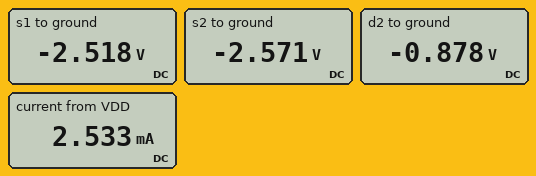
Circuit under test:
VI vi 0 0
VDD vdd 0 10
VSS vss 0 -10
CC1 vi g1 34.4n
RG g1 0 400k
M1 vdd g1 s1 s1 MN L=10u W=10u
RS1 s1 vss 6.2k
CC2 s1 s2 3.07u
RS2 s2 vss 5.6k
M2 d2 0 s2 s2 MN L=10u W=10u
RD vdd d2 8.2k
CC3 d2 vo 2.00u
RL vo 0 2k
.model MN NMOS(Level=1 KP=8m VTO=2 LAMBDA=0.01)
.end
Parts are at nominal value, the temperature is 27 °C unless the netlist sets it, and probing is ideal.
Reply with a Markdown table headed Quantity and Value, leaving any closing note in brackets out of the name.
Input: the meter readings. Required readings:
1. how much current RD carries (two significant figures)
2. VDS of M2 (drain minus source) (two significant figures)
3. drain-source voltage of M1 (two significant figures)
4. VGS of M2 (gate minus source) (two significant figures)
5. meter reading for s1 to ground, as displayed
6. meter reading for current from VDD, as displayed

| Quantity | Value |
|---|---|
| how much current RD carries | 1.3 mA |
| VDS of M2 (drain minus source) | 1.7 V |
| drain-source voltage of M1 | 13 V |
| VGS of M2 (gate minus source) | 2.6 V |
| meter reading for s1 to ground, as displayed | -2.518 V |
| meter reading for current from VDD, as displayed | 2.533 mA |
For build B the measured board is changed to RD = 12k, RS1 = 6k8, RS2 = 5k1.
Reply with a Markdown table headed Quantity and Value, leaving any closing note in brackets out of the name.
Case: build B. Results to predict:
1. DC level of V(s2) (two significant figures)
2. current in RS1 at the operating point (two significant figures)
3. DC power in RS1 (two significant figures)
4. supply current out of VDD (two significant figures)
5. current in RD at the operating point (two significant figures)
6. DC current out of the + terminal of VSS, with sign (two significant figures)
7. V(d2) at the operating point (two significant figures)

| Quantity | Value |
|---|---|
| DC level of V(s2) | -4.1 V |
| current in RS1 at the operating point | 1.1 mA |
| DC power in RS1 | 8.3 mW |
| supply current out of VDD | 2.3 mA |
| current in RD at the operating point | 1.2 mA |
| DC current out of the + terminal of VSS, with sign | -2.3 mA |
| V(d2) at the operating point | -4.0 V |
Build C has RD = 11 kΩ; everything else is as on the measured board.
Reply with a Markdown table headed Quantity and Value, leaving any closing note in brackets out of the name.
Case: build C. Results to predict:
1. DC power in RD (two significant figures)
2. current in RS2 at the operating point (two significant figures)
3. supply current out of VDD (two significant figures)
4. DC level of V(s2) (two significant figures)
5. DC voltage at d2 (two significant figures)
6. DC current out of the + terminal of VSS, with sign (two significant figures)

| Quantity | Value |
|---|---|
| DC power in RD | 16 mW |
| current in RS2 at the operating point | 1.2 mA |
| supply current out of VDD | 2.4 mA |
| DC level of V(s2) | -3.3 V |
| DC voltage at d2 | -3.2 V |
| DC current out of the + terminal of VSS, with sign | -2.4 mA |
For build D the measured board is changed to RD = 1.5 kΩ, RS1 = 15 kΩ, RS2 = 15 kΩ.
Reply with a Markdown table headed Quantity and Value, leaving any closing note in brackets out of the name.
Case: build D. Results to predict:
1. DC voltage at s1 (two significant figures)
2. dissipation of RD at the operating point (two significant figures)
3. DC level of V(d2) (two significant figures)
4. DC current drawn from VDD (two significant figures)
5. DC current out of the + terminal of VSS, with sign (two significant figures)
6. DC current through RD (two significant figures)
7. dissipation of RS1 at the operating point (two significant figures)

| Quantity | Value |
|---|---|
| DC voltage at s1 | -2.3 V |
| dissipation of RD at the operating point | 390 µW |
| DC level of V(d2) | 9.2 V |
| DC current drawn from VDD | 1.0 mA |
| DC current out of the + terminal of VSS, with sign | -1.0 mA |
| DC current through RD | 510 µA |
| dissipation of RS1 at the operating point | 3.9 mW |
